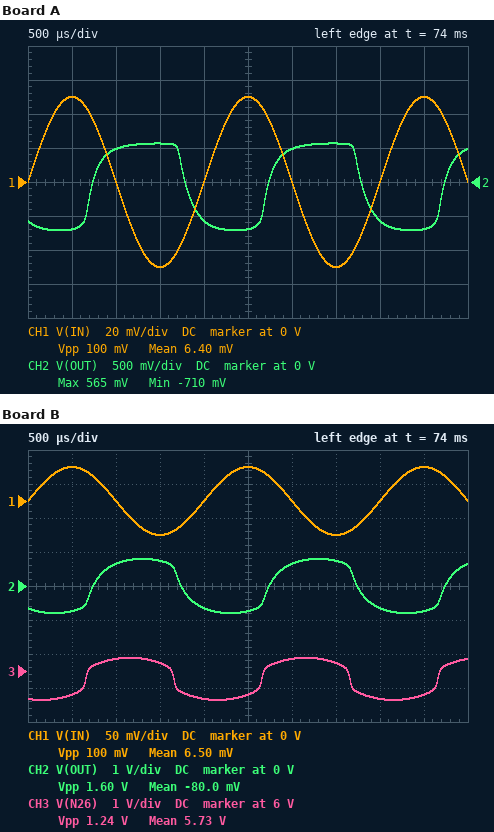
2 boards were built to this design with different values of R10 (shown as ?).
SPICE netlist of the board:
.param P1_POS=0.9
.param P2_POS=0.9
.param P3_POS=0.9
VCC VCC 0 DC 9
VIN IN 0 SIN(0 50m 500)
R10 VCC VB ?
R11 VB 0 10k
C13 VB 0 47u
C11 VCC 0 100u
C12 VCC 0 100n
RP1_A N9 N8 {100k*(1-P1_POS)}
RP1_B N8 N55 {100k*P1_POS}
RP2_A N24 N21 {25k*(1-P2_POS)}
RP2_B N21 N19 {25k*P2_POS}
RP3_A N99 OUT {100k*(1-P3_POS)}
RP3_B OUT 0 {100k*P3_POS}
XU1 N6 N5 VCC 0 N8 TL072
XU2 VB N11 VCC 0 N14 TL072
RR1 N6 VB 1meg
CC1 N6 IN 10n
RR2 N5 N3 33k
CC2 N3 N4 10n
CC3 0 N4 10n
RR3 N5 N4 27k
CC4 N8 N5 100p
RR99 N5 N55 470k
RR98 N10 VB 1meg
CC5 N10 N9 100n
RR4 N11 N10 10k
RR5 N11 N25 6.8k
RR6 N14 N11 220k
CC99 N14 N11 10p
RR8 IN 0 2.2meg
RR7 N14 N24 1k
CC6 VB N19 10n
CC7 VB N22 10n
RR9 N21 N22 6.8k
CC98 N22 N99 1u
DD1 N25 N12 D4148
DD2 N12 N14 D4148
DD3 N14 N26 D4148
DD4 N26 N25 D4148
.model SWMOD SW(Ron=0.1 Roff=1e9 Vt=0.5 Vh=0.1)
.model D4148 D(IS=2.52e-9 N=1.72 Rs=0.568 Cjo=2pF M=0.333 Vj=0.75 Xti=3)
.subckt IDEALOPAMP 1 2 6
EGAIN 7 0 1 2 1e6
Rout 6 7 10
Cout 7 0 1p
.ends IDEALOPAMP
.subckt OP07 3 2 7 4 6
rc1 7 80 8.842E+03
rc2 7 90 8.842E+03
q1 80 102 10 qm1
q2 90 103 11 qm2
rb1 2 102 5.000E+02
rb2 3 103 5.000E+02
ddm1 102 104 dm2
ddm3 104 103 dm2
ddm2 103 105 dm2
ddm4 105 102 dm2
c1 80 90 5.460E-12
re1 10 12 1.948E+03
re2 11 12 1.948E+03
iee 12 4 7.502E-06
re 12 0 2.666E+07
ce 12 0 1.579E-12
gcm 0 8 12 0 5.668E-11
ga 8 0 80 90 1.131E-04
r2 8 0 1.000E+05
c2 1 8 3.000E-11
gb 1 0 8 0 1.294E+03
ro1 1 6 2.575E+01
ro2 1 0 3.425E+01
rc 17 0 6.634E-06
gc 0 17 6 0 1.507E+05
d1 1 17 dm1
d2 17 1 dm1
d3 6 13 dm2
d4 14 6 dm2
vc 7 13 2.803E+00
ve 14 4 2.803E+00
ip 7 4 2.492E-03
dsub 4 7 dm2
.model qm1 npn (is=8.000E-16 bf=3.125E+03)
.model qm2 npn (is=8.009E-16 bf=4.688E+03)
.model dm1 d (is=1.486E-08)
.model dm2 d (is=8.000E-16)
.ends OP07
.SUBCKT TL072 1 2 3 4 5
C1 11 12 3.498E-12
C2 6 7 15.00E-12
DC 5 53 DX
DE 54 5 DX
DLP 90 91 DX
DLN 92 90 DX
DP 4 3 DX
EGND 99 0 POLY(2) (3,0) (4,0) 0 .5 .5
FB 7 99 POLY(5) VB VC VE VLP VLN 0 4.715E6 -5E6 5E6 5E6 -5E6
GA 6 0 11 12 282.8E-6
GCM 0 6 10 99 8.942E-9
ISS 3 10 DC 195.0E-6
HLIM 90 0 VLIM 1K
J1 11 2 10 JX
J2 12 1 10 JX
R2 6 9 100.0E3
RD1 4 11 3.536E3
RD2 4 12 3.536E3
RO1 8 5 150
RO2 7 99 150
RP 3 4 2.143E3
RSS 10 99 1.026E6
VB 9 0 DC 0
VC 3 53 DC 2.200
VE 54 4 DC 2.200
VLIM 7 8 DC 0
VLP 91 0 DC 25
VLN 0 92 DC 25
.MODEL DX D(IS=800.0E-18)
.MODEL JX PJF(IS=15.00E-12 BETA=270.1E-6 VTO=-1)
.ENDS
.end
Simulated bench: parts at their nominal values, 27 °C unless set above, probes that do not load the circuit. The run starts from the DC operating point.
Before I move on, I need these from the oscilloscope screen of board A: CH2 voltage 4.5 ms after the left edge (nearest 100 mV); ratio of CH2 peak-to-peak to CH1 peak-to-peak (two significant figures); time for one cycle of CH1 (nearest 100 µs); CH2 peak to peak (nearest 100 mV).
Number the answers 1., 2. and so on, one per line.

1. -700 mV
2. 13
3. 2.0 ms
4. 1.3 V
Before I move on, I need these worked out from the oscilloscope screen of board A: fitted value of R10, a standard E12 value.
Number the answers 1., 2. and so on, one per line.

1. 3.3 kΩ
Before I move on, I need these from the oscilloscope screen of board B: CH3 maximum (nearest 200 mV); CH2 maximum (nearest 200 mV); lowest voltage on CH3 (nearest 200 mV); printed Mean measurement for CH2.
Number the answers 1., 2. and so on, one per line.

1. 6.4 V
2. 800 mV
3. 5.2 V
4. -80.0 mV
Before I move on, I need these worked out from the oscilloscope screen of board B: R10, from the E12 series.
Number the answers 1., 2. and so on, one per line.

1. 5.6 kΩ
